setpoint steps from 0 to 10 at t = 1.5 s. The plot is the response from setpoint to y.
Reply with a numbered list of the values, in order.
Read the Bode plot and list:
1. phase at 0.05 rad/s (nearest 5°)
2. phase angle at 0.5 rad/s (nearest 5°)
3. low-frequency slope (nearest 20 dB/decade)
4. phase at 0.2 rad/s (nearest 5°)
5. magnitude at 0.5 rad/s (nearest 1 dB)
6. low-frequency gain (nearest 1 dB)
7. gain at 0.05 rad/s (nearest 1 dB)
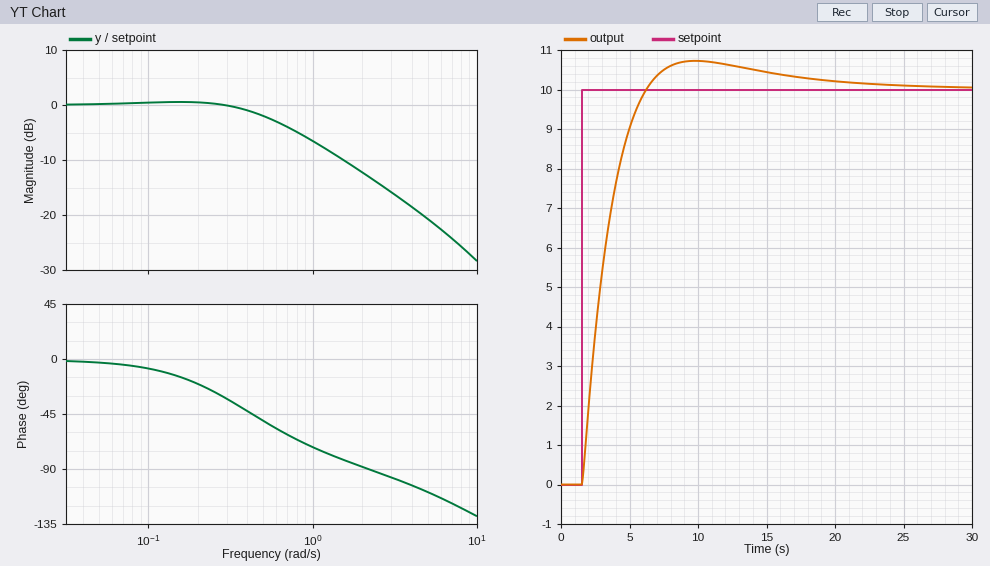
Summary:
1. -5°
2. -50°
3. 0 dB/decade
4. -20°
5. -2 dB
6. 0 dB
7. 0 dB
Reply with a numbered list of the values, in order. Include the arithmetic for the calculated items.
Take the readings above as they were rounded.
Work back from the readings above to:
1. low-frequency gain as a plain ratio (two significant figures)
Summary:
1. 10^(0 / 20) = 1.0
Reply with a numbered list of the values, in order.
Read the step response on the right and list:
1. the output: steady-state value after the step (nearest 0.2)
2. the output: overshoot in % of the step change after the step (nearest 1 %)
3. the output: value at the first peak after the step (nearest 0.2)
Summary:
1. 10.0
2. 7 %
3. 10.8
